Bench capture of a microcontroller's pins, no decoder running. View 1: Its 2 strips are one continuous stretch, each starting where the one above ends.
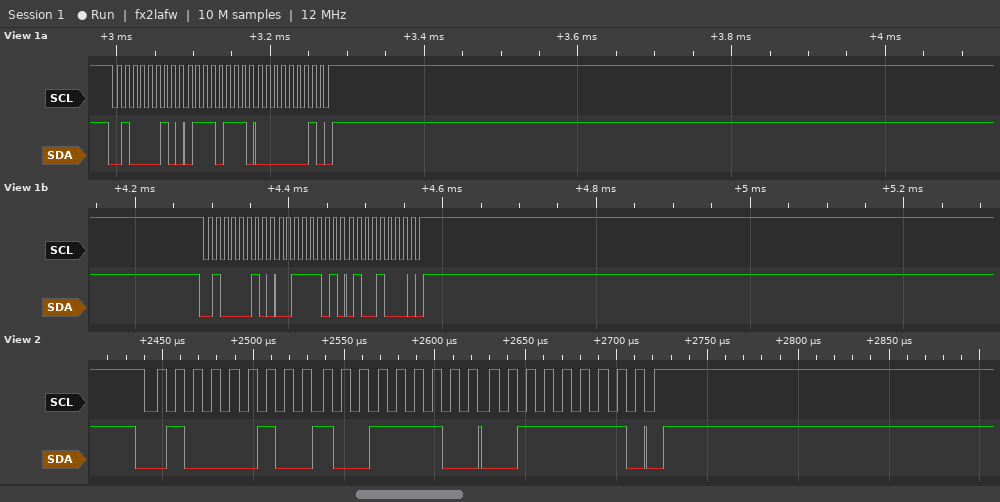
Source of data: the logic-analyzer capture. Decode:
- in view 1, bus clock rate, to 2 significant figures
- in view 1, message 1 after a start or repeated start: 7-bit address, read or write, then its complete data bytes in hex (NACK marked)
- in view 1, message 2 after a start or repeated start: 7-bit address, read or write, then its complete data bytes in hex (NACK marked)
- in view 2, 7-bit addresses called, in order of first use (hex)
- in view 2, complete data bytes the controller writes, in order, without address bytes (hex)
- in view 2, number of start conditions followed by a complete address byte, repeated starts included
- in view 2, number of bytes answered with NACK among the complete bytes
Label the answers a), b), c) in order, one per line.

a) 100 kHz
b) 0x21 write: 77 01
c) 0x21 write: 3D 48
d) 0x21
e) 9E 3F
f) 1
g) 0
